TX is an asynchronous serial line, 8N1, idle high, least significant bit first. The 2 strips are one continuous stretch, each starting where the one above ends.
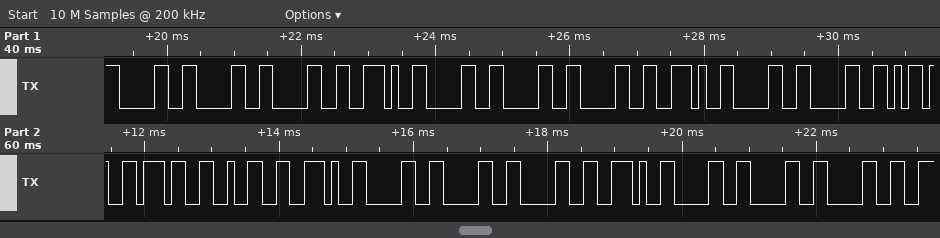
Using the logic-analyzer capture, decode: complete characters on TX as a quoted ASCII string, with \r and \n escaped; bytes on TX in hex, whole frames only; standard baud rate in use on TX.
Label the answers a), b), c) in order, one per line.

a) "000.000.00-72.000.000"
b) 0x30 0x30 0x30 0x2E 0x30 0x30 0x30 0x2E 0x30 0x30 0x2D 0x37 0x32 0x2E 0x30 0x30 0x30 0x2E 0x30 0x30 0x30
c) 9600 baud
